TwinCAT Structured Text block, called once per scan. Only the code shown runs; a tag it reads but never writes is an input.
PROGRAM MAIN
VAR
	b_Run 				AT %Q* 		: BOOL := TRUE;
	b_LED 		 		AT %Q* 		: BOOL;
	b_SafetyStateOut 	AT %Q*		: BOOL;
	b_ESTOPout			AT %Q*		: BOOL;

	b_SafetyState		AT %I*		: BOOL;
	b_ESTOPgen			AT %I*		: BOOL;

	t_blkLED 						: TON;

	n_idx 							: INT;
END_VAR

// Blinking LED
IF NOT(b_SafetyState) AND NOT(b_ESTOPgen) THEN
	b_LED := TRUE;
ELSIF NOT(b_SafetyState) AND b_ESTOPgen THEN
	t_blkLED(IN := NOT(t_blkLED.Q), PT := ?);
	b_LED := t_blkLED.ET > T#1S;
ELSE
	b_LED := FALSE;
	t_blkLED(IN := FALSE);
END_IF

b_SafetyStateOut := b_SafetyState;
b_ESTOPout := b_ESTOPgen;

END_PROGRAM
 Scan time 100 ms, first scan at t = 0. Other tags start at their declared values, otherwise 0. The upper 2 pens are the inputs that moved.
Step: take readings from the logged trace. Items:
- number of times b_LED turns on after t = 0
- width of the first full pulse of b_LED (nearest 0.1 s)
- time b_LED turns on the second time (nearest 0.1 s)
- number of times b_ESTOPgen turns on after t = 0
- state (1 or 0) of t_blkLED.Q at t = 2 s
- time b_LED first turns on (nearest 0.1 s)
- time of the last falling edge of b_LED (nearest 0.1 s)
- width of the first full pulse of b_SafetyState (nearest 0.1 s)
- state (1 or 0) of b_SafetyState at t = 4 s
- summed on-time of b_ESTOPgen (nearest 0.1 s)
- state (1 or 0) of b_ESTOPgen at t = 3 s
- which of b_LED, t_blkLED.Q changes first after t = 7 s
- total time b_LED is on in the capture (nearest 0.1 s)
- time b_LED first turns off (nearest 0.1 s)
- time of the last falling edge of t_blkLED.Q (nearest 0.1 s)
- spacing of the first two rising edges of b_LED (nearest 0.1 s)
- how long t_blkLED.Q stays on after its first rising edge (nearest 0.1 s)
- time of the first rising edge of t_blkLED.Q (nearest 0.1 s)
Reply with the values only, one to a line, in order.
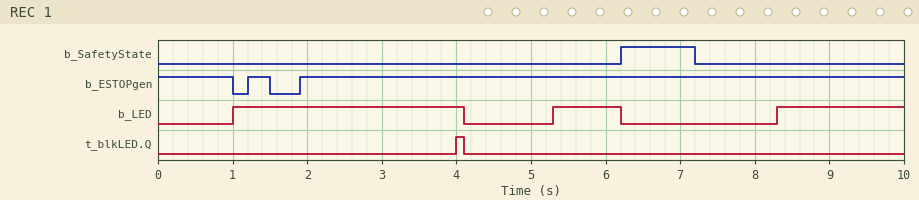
3
3.1 s
5.3 s
2
0
1.0 s
6.2 s
1.0 s
0
9.4 s
1
b_LED
5.7 s
4.1 s
4.1 s
4.3 s
0.1 s
4.0 s
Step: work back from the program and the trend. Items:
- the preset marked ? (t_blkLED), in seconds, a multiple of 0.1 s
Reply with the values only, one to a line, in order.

4.0 s
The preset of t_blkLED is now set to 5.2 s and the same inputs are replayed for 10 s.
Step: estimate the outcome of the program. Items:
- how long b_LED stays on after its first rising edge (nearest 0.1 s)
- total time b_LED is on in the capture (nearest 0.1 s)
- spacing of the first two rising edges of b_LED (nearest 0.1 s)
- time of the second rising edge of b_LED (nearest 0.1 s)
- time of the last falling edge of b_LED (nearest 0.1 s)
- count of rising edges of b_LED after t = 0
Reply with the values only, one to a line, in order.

4.3 s
6.0 s
7.3 s
8.3 s
5.3 s
2
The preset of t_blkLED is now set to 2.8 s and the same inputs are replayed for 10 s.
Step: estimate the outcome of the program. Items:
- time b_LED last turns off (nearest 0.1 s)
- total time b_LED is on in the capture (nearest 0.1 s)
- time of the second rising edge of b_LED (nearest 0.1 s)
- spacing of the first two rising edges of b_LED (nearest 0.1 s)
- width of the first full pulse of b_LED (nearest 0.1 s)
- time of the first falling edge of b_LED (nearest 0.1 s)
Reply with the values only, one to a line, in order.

5.9 s
5.4 s
4.1 s
3.1 s
1.9 s
2.9 s
